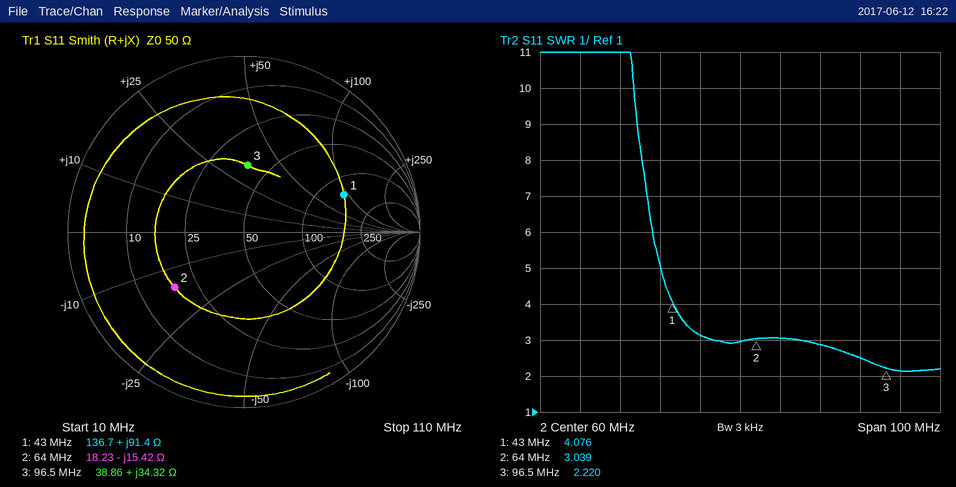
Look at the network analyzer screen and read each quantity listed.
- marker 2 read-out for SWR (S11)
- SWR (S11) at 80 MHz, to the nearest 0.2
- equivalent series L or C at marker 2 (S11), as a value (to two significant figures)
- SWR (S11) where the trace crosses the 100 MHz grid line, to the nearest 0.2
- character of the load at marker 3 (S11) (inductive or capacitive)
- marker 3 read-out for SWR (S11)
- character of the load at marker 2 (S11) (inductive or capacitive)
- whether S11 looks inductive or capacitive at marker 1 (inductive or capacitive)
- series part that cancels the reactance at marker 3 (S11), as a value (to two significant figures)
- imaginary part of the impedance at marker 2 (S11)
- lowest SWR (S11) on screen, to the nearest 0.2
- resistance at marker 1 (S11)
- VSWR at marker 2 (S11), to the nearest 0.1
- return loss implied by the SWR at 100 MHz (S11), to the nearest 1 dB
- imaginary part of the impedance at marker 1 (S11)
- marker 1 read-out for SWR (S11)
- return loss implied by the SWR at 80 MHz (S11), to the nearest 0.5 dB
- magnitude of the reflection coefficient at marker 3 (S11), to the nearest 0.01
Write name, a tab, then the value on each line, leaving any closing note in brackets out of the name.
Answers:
marker 2 read-out for SWR	3.039
SWR (S11) at 80 MHz, to the nearest 0.2	2.8
equivalent series L or C at marker 2 (S11), as a value	160 pF
SWR (S11) where the trace crosses the 100 MHz grid line, to the nearest 0.2	2.2
character of the load at marker 3 (S11)	inductive
marker 3 read-out for SWR	2.220
character of the load at marker 2 (S11)	capacitive
whether S11 looks inductive or capacitive at marker 1	inductive
series part that cancels the reactance at marker 3 (S11), as a value	48 pF
imaginary part of the impedance at marker 2	-15.42 Ω
lowest SWR (S11) on screen, to the nearest 0.2	2.2
resistance at marker 1	136.7 Ω
VSWR at marker 2 (S11), to the nearest 0.1	3.0
return loss implied by the SWR at 100 MHz (S11), to the nearest 1 dB	9 dB
imaginary part of the impedance at marker 1	+91.4 Ω
marker 1 read-out for SWR	4.076
return loss implied by the SWR at 80 MHz (S11), to the nearest 0.5 dB	6.5 dB
magnitude of the reflection coefficient at marker 3 (S11), to the nearest 0.01	0.38
